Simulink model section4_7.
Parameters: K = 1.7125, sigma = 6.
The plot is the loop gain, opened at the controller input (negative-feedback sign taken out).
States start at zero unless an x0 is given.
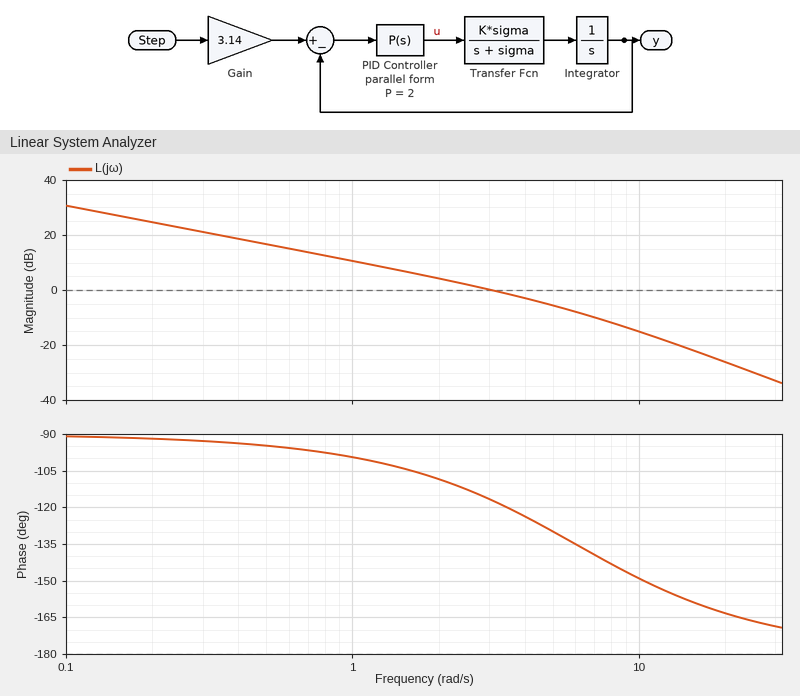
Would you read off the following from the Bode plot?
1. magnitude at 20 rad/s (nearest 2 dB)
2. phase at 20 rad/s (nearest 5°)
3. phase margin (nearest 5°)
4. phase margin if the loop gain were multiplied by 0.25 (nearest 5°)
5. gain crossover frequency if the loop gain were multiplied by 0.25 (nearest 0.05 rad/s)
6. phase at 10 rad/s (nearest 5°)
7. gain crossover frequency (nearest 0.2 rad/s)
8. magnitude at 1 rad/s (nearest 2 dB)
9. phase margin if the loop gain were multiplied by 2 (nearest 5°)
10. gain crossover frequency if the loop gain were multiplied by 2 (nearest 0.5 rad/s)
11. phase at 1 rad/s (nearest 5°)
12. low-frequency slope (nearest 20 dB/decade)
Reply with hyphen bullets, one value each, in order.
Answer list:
- -26 dB
- -165°
- 65°
- 80°
- 0.85 rad/s
- -150°
- 3.0 rad/s
- 10 dB
- 50°
- 5.0 rad/s
- -100°
- -20 dB/decade
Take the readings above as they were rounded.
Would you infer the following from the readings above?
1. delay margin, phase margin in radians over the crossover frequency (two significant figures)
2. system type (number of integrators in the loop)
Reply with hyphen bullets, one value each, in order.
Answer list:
- 0.38 s
- 1
